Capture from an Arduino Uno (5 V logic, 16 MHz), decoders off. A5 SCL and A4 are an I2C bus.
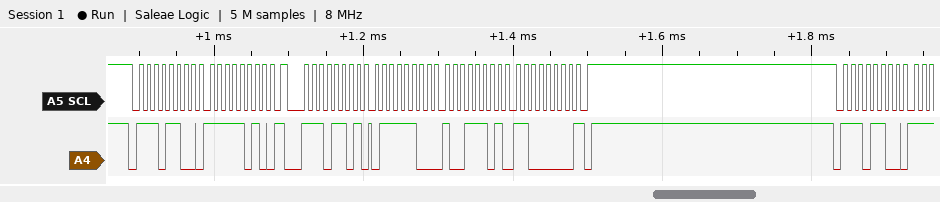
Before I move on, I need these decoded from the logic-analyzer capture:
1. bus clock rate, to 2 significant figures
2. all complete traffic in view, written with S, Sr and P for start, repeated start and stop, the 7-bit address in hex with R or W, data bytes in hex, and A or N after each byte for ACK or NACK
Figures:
100 kHz
S 76W A FA A Sr 76R A 7C A 9D A C0 N P S 76W A
